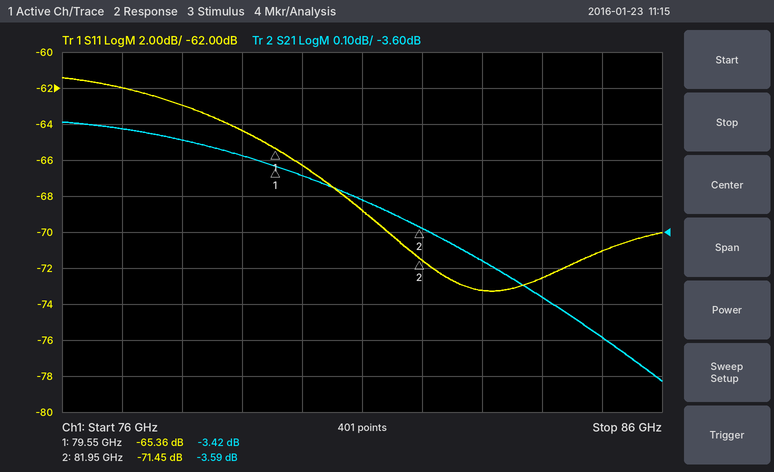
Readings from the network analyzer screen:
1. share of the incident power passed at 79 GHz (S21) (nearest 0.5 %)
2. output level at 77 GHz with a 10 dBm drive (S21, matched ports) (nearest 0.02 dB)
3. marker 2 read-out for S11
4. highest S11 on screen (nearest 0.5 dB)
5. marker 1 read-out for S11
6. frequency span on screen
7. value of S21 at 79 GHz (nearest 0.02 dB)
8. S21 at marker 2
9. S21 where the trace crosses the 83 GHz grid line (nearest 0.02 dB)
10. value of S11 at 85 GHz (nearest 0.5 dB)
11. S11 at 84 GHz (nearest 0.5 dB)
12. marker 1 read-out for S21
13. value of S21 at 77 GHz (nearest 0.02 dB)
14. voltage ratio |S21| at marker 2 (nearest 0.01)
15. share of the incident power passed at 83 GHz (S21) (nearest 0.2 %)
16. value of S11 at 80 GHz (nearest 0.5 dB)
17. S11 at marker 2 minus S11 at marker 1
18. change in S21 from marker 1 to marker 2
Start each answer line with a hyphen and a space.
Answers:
- 46.0 %
- 6.68 dBm
- -71.45 dB
- -61.5 dB
- -65.36 dB
- 10 GHz
- -3.38 dB
- -3.59 dB
- -3.68 dB
- -71.0 dB
- -72.5 dB
- -3.42 dB
- -3.32 dB
- 0.66
- 42.8 %
- -66.5 dB
- -6.09 dB
- -0.17 dB
